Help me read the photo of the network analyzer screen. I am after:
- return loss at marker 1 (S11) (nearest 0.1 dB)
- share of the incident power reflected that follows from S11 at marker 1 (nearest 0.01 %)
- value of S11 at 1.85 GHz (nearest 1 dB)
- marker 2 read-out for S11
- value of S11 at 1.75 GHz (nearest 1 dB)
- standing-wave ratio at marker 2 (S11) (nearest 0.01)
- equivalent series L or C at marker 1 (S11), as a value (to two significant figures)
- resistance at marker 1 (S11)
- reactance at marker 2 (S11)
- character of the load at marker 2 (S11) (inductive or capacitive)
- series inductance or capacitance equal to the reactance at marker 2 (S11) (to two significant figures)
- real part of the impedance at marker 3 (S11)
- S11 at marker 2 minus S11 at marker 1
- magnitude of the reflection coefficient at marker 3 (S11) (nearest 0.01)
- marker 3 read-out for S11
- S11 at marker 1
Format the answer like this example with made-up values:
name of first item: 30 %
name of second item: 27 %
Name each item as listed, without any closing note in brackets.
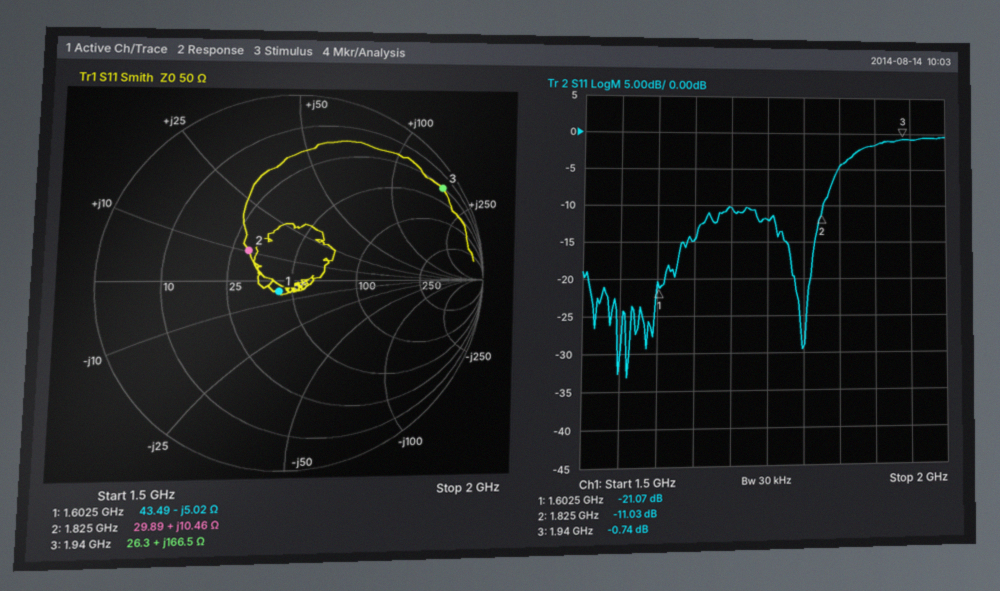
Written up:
return loss at marker 1 (S11): 21.1 dB
share of the incident power reflected that follows from S11 at marker 1: 0.78 %
value of S11 at 1.85 GHz: -5 dB
marker 2 read-out for S11: -11.03 dB
value of S11 at 1.75 GHz: -12 dB
standing-wave ratio at marker 2 (S11): 1.78
equivalent series L or C at marker 1 (S11), as a value: 20 pF
resistance at marker 1: 43.49 Ω
reactance at marker 2: +10.46 Ω
character of the load at marker 2 (S11): inductive
series inductance or capacitance equal to the reactance at marker 2 (S11): 910 pH
real part of the impedance at marker 3: 26.3 Ω
S11 at marker 2 minus S11 at marker 1: 10.04 dB
magnitude of the reflection coefficient at marker 3 (S11): 0.92
marker 3 read-out for S11: -0.74 dB
S11 at marker 1: -21.07 dB
